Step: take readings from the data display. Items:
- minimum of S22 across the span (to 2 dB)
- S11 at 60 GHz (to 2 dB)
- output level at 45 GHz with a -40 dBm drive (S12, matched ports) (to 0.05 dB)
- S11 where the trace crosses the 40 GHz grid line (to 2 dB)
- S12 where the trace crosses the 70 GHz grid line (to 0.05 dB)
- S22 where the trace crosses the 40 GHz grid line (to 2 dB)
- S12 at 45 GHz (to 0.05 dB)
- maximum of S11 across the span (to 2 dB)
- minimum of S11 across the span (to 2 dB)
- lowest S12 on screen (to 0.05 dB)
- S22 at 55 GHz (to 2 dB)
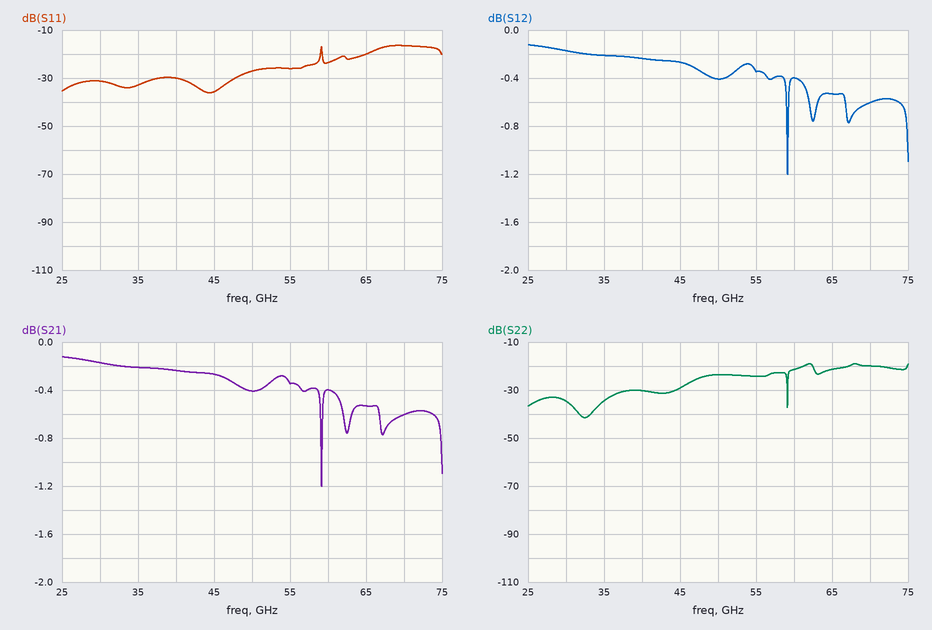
-42 dB
-24 dB
-40.25 dBm
-30 dB
-0.60 dB
-30 dB
-0.25 dB
-16 dB
-36 dB
-1.20 dB
-24 dB
